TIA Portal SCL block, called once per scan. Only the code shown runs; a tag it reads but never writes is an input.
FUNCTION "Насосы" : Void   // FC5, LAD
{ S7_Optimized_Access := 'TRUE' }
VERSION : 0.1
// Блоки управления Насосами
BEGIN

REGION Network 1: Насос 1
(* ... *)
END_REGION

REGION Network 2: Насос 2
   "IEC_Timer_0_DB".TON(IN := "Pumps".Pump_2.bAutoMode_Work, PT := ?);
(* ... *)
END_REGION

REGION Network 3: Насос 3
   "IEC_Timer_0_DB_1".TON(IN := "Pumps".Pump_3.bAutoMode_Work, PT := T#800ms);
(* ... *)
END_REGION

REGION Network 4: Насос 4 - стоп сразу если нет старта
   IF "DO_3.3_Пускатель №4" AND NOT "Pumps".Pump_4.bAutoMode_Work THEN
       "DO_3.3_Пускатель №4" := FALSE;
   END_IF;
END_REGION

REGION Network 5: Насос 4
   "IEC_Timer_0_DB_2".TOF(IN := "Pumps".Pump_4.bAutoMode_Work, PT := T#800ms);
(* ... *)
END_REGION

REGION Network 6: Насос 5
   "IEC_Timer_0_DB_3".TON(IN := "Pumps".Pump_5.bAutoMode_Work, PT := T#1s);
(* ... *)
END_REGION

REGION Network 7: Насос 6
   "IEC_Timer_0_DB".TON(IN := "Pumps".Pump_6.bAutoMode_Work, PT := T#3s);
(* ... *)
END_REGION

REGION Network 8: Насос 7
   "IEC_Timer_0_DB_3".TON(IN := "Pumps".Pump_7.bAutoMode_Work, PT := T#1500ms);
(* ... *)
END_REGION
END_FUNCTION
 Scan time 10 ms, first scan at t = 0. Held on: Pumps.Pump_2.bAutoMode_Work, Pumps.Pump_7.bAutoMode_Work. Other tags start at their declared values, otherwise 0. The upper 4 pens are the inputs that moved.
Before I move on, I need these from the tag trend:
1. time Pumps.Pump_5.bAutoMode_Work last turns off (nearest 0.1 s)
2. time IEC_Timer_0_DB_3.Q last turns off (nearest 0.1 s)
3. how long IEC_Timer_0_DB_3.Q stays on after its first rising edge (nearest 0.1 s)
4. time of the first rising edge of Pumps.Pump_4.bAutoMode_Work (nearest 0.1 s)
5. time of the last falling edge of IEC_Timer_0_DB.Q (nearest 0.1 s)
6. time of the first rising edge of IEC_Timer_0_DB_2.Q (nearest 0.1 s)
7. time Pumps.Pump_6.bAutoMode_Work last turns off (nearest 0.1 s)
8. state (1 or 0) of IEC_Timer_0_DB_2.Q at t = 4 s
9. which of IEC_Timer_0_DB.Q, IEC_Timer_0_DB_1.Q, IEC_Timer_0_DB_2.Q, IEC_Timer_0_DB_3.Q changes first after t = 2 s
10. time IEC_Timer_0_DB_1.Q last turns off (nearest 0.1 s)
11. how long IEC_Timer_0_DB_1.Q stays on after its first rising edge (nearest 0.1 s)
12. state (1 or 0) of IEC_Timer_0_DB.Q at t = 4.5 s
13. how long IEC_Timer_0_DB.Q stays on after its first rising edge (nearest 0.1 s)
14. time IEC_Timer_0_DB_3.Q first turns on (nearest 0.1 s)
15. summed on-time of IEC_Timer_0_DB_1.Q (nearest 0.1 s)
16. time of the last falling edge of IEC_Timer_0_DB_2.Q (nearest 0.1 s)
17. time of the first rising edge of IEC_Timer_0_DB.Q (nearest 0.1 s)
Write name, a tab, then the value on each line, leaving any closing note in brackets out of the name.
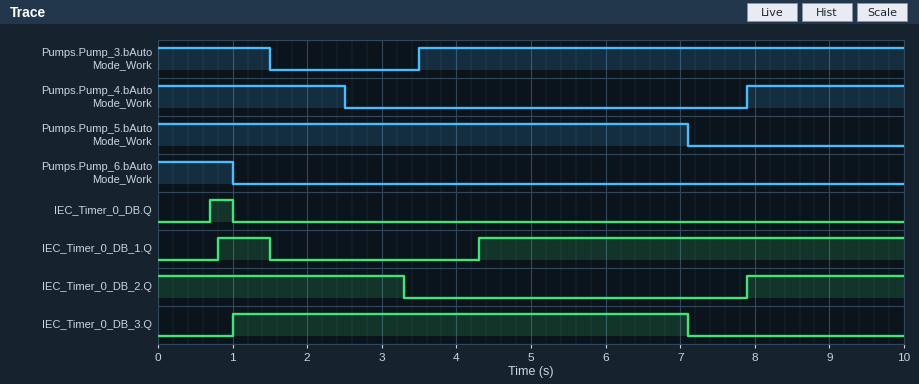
time Pumps.Pump_5.bAutoMode_Work last turns off	7.1 s
time IEC_Timer_0_DB_3.Q last turns off	7.1 s
how long IEC_Timer_0_DB_3.Q stays on after its first rising edge	6.1 s
time of the first rising edge of Pumps.Pump_4.bAutoMode_Work	7.9 s
time of the last falling edge of IEC_Timer_0_DB.Q	1.0 s
time of the first rising edge of IEC_Timer_0_DB_2.Q	7.9 s
time Pumps.Pump_6.bAutoMode_Work last turns off	1.0 s
state (1 or 0) of IEC_Timer_0_DB_2.Q at t = 4 s	0
which of IEC_Timer_0_DB.Q, IEC_Timer_0_DB_1.Q, IEC_Timer_0_DB_2.Q, IEC_Timer_0_DB_3.Q changes first after t = 2 s	IEC_Timer_0_DB_2.Q
time IEC_Timer_0_DB_1.Q last turns off	1.5 s
how long IEC_Timer_0_DB_1.Q stays on after its first rising edge	0.7 s
state (1 or 0) of IEC_Timer_0_DB.Q at t = 4.5 s	0
how long IEC_Timer_0_DB.Q stays on after its first rising edge	0.3 s
time IEC_Timer_0_DB_3.Q first turns on	1.0 s
summed on-time of IEC_Timer_0_DB_1.Q	6.4 s
time of the last falling edge of IEC_Timer_0_DB_2.Q	3.3 s
time of the first rising edge of IEC_Timer_0_DB.Q	0.7 s
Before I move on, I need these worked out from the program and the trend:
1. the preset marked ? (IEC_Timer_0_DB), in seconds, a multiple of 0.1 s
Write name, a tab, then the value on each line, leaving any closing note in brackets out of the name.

the preset marked ? (IEC_Timer_0_DB), in seconds, a multiple of 0.1 s	0.7 s
